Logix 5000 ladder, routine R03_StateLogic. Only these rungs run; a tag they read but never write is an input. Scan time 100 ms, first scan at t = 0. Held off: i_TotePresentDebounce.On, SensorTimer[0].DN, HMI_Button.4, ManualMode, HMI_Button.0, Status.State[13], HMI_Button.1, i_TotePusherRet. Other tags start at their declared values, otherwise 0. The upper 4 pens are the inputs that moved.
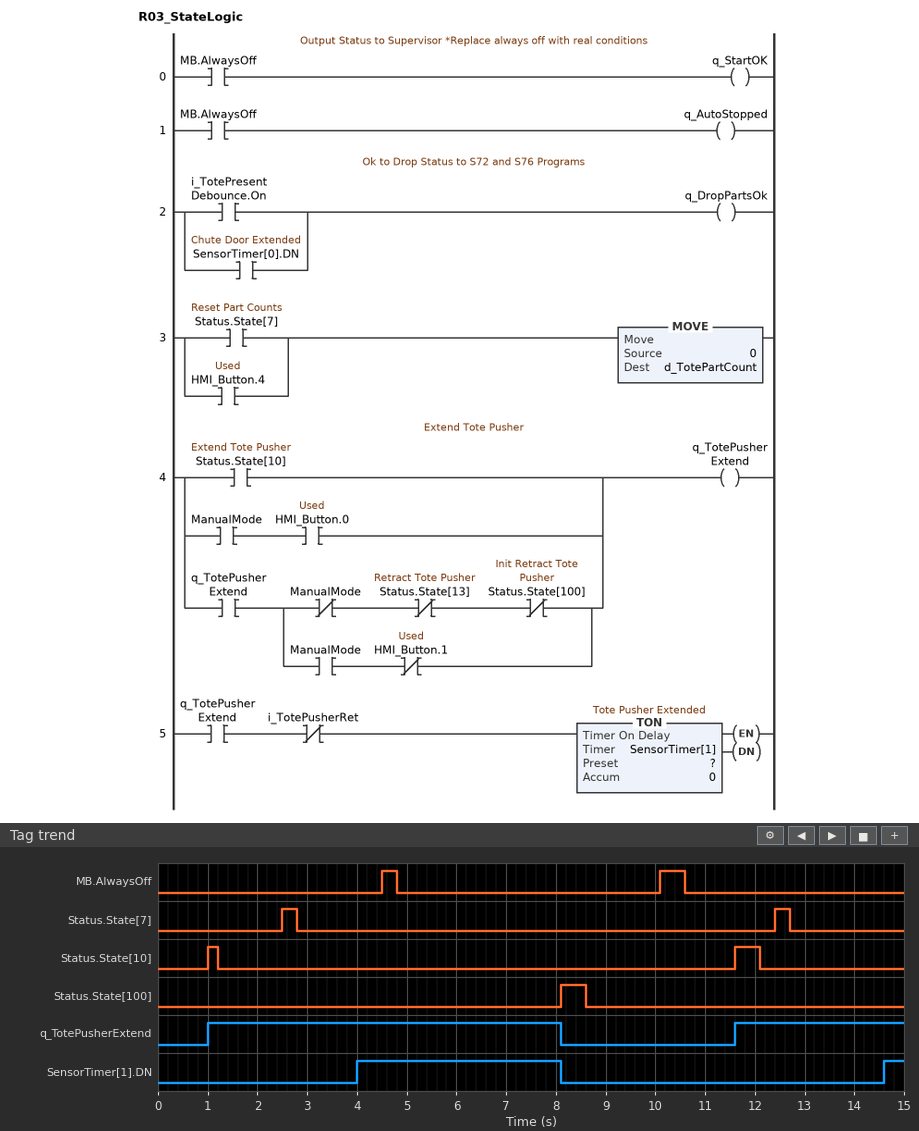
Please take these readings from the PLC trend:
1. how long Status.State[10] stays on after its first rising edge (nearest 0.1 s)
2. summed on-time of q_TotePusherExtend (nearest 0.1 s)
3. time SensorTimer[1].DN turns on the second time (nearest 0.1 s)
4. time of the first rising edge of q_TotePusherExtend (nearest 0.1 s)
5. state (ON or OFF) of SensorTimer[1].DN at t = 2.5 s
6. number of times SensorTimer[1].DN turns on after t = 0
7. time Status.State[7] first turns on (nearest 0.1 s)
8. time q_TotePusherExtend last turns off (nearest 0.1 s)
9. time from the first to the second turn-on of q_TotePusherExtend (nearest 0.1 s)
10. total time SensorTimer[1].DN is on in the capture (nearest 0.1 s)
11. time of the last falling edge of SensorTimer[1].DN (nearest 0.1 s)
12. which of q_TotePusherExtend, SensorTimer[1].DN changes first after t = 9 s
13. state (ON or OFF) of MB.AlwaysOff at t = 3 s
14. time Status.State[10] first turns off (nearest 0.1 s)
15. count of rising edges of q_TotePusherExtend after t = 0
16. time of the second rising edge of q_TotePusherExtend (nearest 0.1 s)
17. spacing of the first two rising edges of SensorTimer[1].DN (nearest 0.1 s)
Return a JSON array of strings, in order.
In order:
["0.2 s", "10.5 s", "14.6 s", "1.0 s", "OFF", "2", "2.5 s", "8.1 s", "10.6 s", "4.5 s", "8.1 s", "q_TotePusherExtend", "OFF", "1.2 s", "2", "11.6 s", "10.6 s"]
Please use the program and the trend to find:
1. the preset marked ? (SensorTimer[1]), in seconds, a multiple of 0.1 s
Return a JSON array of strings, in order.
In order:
["3.0 s"]
